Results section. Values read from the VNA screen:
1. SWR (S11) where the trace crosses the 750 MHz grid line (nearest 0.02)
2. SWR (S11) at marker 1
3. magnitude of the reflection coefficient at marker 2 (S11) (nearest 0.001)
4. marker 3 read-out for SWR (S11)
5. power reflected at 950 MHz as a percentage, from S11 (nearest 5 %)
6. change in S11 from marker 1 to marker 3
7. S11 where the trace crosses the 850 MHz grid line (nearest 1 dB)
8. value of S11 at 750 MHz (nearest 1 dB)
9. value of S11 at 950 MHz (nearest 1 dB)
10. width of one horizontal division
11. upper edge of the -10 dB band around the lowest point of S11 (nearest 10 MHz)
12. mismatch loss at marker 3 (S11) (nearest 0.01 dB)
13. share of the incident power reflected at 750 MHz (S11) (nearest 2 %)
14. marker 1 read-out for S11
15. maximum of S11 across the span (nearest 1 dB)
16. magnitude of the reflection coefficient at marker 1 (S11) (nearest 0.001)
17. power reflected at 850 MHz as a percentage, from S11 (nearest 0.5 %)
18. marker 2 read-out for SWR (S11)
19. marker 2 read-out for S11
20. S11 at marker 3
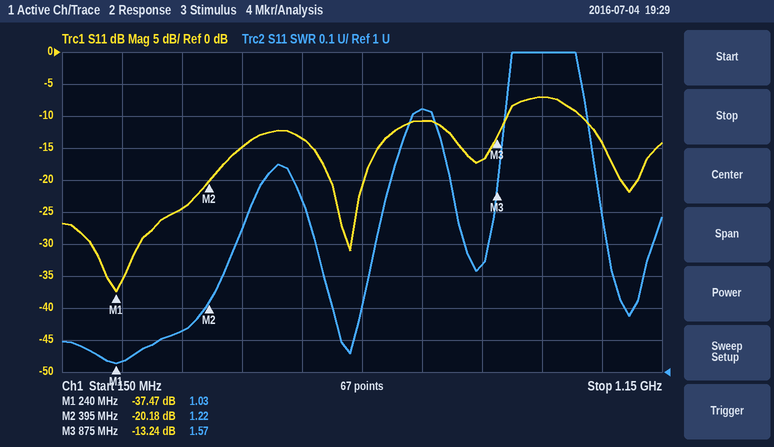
1.82
1.03
0.098
1.57
20 %
24.23 dB
-17 dB
-11 dB
-7 dB
100 MHz
890 MHz
0.21 dB
8 %
-37.47 dB
-7 dB
0.013
2.0 %
1.22
-20.18 dB
-13.24 dB
